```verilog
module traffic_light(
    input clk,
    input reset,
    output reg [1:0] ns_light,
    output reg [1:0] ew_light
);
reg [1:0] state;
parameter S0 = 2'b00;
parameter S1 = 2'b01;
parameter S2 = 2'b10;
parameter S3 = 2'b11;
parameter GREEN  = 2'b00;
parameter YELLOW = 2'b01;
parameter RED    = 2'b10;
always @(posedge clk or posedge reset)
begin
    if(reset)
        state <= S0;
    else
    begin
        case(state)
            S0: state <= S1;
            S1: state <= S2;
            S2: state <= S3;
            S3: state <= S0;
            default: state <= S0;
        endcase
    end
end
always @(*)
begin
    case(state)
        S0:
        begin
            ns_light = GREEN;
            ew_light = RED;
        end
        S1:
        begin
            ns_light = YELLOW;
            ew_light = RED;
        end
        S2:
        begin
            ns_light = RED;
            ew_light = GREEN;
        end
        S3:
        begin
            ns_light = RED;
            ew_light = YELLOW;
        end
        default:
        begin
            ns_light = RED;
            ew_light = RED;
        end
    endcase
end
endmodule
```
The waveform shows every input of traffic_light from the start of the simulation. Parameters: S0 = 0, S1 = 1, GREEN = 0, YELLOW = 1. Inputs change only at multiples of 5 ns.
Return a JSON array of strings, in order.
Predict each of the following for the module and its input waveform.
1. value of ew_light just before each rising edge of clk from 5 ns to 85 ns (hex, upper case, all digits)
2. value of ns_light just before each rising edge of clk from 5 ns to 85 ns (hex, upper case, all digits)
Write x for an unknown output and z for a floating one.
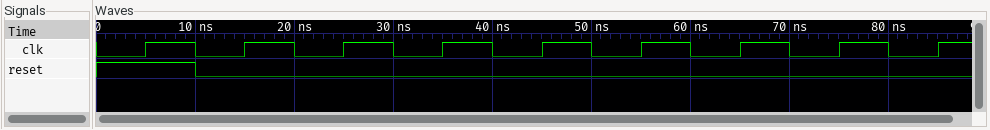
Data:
["2, 2, 2, 0, 1, 2, 2, 0, 1", "0, 0, 1, 2, 2, 0, 1, 2, 2"]
